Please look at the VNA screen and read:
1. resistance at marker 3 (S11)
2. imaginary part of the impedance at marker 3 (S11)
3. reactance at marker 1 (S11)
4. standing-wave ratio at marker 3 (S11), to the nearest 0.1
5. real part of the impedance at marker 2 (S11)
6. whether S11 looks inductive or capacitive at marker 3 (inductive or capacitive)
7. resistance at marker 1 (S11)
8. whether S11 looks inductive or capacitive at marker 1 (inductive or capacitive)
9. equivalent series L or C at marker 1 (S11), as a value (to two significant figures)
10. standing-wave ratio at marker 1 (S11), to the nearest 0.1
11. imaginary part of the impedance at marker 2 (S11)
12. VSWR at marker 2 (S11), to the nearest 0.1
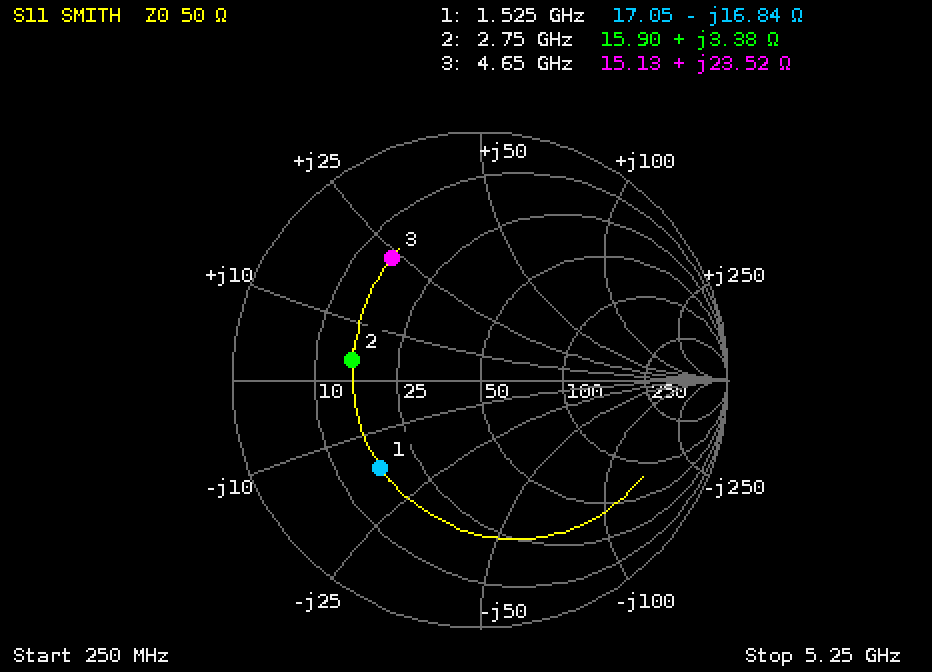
15.13 Ω
+23.52 Ω
-16.84 Ω
4.1
15.90 Ω
inductive
17.05 Ω
capacitive
6.2 pF
3.3
+3.38 Ω
3.2
